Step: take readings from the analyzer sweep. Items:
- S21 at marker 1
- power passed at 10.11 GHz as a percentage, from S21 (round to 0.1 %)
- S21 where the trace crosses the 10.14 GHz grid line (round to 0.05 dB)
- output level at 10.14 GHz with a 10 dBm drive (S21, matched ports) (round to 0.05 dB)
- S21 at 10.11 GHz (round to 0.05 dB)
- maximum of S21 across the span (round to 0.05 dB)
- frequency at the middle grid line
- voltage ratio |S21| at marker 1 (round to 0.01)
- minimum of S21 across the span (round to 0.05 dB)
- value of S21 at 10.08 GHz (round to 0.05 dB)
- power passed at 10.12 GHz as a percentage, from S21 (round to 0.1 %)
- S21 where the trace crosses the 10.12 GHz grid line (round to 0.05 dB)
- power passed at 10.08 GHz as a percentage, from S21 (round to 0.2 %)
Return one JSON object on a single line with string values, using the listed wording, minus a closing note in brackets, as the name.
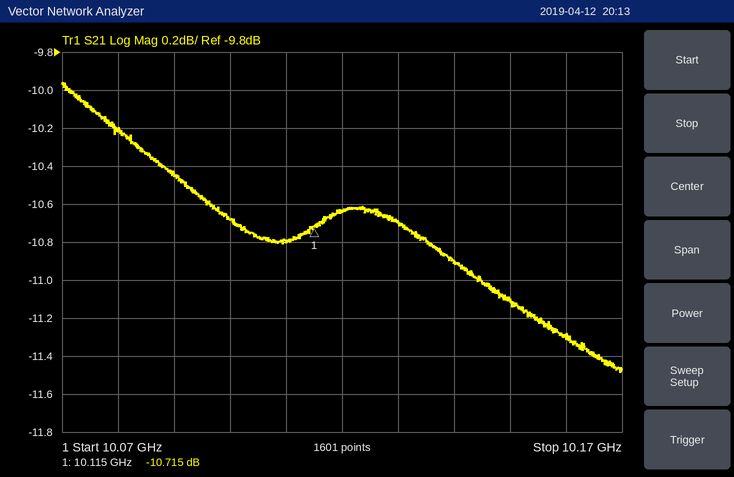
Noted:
{"S21 at marker 1": "-10.715 dB", "power passed at 10.11 GHz as a percentage, from S21": "8.3 %", "S21 where the trace crosses the 10.14 GHz grid line": "-10.90 dB", "output level at 10.14 GHz with a 10 dBm drive (S21, matched ports)": "-0.90 dBm", "S21 at 10.11 GHz": "-10.80 dB", "maximum of S21 across the span": "-9.95 dB", "frequency at the middle grid line": "10.12 GHz", "voltage ratio |S21| at marker 1": "0.29", "minimum of S21 across the span": "-11.50 dB", "value of S21 at 10.08 GHz": "-10.20 dB", "power passed at 10.12 GHz as a percentage, from S21": "8.6 %", "S21 where the trace crosses the 10.12 GHz grid line": "-10.65 dB", "power passed at 10.08 GHz as a percentage, from S21": "9.6 %"}
